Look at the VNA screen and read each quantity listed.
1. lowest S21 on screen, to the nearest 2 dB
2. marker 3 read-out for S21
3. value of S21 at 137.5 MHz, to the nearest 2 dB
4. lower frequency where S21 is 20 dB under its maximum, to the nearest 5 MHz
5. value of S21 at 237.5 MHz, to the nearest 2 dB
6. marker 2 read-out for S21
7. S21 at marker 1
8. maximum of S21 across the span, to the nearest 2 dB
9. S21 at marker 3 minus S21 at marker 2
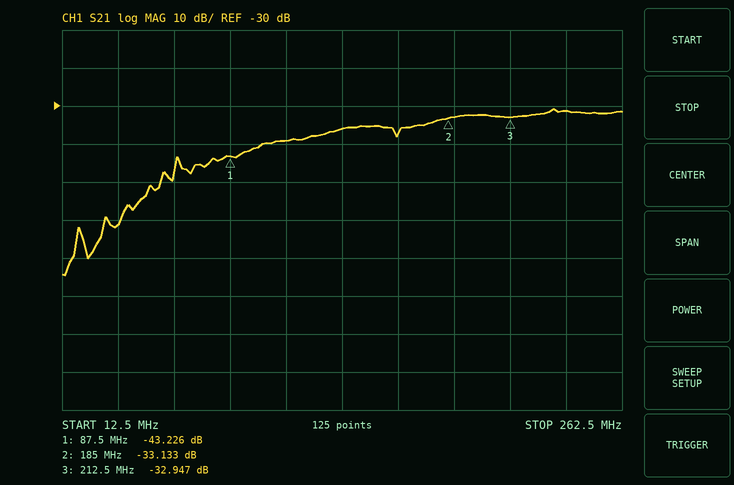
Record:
-74 dB
-32.947 dB
-36 dB
55 MHz
-32 dB
-33.133 dB
-43.226 dB
-30 dB
0.186 dB
